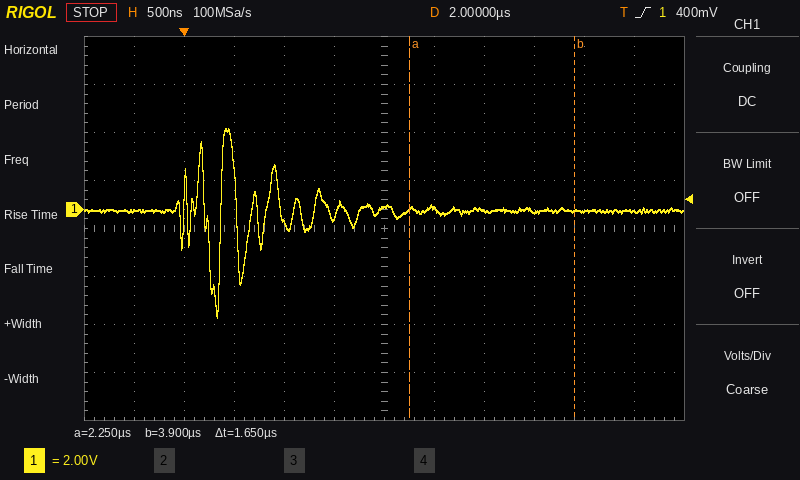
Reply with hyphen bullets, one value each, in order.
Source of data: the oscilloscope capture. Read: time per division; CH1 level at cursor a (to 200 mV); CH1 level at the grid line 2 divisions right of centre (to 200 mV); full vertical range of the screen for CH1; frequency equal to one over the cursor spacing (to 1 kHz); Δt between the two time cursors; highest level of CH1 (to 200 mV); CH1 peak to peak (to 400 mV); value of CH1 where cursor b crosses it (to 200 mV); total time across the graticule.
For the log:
- 500 ns
- 0.0 V
- 0.0 V
- 16 V
- 606 kHz
- 1.65 µs
- 3.4 V
- 8.0 V
- 0.0 V
- 6 µs
